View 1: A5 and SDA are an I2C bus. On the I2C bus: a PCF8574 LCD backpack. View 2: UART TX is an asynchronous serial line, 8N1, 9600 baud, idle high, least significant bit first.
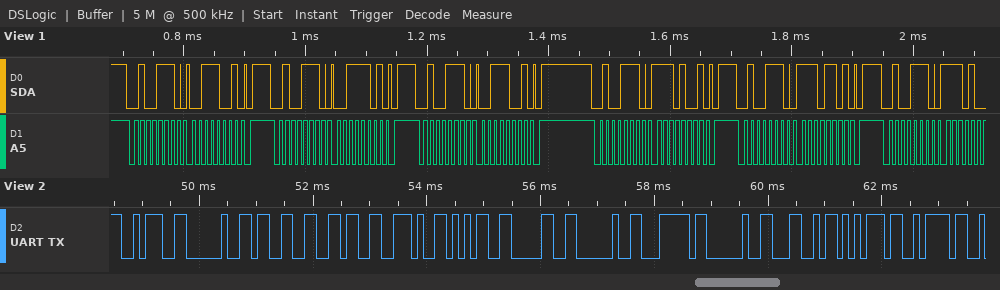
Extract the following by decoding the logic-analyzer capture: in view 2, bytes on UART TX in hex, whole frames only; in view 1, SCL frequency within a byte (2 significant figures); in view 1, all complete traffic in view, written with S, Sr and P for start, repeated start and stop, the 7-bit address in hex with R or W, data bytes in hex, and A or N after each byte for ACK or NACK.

3A 20 33 36 2E 35 30 20 7C 20 4C 75 7A
100 kHz
S 27W A 39 A P S 27W A 3D A P S 27W A 39 A P S 27W A E9 A P S 27W A ED A P S 27W A
